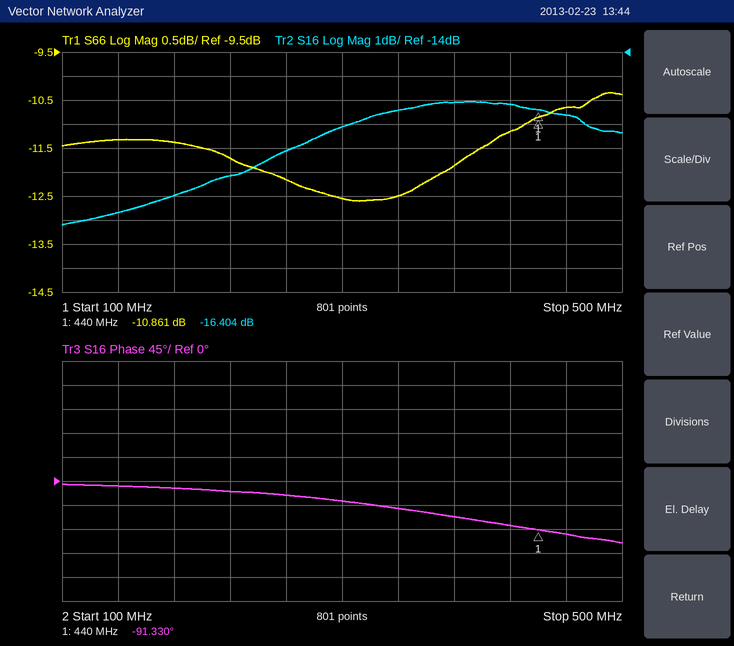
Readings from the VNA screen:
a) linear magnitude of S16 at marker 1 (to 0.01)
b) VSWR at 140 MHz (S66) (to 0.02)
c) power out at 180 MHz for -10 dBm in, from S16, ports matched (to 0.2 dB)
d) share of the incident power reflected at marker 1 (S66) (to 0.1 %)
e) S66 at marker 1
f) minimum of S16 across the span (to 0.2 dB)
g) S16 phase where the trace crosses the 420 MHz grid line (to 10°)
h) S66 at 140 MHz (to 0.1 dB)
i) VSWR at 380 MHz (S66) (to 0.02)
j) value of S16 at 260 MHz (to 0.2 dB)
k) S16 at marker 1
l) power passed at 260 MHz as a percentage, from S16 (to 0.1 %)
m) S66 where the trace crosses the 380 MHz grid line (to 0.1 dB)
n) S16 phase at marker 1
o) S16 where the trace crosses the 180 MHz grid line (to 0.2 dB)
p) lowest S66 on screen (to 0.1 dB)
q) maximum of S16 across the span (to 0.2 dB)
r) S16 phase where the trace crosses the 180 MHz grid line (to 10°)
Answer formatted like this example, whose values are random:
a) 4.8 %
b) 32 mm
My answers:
a) 0.15
b) 1.74
c) -30.0 dBm
d) 8.2 %
e) -10.861 dB
f) -21.2 dB
g) -80°
h) -11.3 dB
i) 1.68
j) -18.2 dB
k) -16.404 dB
l) 1.5 %
m) -11.9 dB
n) -91.330°
o) -20.0 dB
p) -12.6 dB
q) -16.0 dB
r) -10°
